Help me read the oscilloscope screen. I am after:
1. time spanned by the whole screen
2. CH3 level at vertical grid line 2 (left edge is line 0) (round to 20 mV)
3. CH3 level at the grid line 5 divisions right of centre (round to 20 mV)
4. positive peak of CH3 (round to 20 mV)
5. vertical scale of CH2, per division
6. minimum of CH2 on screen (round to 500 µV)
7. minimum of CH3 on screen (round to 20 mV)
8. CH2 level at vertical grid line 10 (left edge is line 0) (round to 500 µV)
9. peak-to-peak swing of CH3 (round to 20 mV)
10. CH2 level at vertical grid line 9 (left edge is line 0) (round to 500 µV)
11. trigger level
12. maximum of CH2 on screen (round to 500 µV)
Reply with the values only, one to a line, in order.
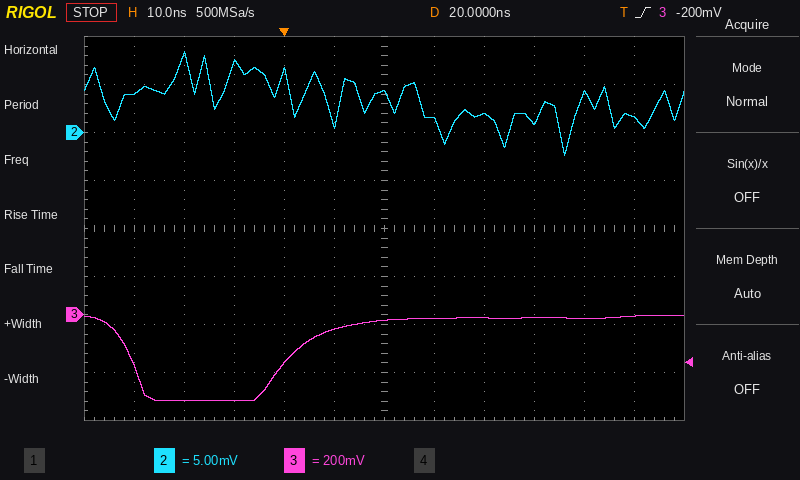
120 ns
-360 mV
0 mV
0 mV
5 mV
-2.5 mV
-360 mV
4.0 mV
360 mV
1.0 mV
-200 mV
8.5 mV
